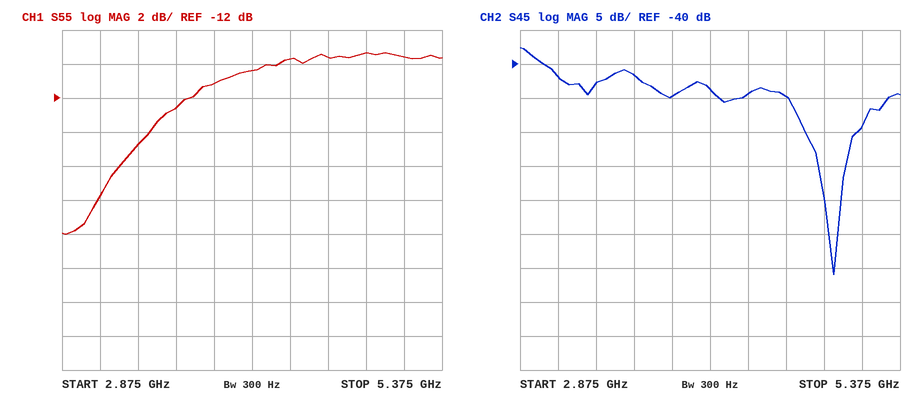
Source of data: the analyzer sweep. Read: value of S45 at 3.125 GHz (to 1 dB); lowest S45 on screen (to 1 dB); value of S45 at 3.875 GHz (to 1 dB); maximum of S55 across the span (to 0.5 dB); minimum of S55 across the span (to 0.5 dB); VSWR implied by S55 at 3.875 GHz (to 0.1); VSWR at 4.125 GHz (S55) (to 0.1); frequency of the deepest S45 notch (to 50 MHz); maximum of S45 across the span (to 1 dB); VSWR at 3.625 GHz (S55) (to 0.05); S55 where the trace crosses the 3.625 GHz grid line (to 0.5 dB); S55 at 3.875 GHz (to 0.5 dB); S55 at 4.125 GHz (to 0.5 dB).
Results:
-42 dB
-71 dB
-45 dB
-9.5 dB
-20.0 dB
1.8
1.9
4.95 GHz
-38 dB
1.60
-12.5 dB
-11.0 dB
-10.5 dB
